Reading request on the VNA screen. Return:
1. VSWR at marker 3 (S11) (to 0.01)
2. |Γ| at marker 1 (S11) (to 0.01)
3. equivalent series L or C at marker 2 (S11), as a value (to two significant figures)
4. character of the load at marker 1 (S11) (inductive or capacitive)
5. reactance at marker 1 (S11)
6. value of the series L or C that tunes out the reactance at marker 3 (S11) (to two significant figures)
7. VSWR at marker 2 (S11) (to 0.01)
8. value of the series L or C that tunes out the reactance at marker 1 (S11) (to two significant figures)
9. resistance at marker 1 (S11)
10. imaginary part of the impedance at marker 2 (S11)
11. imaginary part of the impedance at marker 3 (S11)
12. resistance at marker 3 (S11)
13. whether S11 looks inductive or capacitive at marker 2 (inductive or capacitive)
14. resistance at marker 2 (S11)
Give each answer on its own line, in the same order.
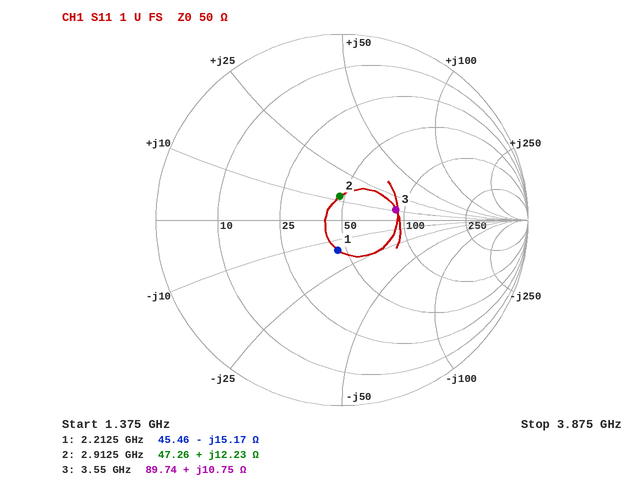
1.83
0.16
670 pH
capacitive
-15.17 Ω
4.2 pF
1.29
1.1 nH
45.46 Ω
+12.23 Ω
+10.75 Ω
89.74 Ω
inductive
47.26 Ω
